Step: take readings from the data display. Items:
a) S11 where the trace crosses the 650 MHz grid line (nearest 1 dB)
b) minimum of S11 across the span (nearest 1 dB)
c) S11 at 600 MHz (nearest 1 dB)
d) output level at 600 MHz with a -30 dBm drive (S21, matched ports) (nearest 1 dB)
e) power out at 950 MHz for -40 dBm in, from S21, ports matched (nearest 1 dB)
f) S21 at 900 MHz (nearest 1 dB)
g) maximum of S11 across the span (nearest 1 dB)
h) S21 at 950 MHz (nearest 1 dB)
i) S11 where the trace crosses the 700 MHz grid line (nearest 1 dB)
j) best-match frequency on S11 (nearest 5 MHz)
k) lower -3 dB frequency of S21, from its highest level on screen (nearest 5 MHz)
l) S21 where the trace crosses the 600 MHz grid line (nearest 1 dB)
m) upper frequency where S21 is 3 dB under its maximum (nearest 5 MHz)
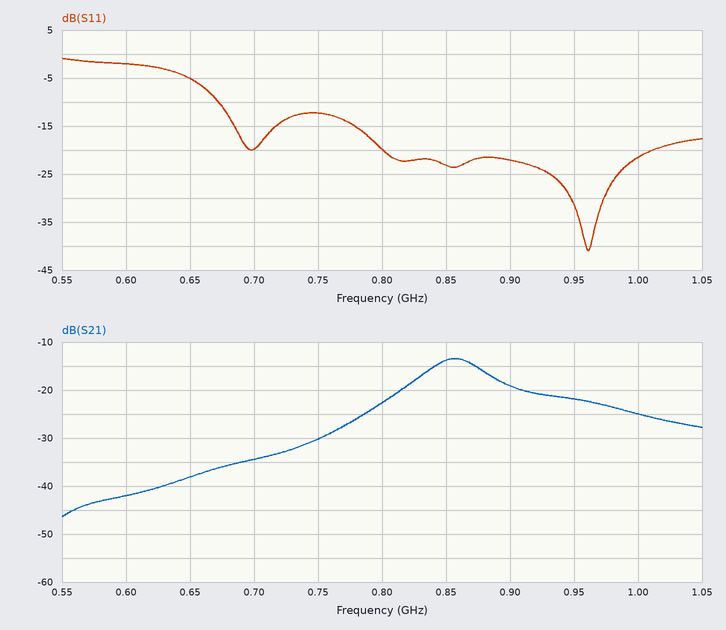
-5 dB
-41 dB
-2 dB
-72 dBm
-62 dBm
-19 dB
-1 dB
-22 dB
-20 dB
960 MHz
835 MHz
-42 dB
880 MHz
